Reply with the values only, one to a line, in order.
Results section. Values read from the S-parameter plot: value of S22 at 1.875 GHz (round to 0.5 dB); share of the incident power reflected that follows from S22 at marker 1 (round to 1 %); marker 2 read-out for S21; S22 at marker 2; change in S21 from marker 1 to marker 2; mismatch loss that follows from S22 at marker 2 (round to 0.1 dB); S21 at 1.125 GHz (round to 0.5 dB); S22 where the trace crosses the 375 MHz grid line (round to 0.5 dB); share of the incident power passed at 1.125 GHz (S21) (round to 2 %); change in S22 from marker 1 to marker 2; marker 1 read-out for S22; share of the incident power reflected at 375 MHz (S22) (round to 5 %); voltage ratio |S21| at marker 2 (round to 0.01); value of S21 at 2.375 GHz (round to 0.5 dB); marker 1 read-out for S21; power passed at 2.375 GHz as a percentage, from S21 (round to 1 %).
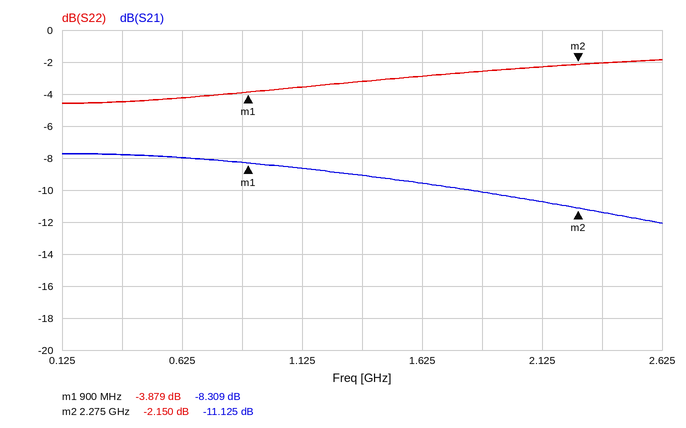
-2.5 dB
41 %
-11.125 dB
-2.150 dB
-2.816 dB
4.1 dB
-8.5 dB
-4.5 dB
14 %
1.729 dB
-3.879 dB
35 %
0.28
-11.5 dB
-8.309 dB
7 %
